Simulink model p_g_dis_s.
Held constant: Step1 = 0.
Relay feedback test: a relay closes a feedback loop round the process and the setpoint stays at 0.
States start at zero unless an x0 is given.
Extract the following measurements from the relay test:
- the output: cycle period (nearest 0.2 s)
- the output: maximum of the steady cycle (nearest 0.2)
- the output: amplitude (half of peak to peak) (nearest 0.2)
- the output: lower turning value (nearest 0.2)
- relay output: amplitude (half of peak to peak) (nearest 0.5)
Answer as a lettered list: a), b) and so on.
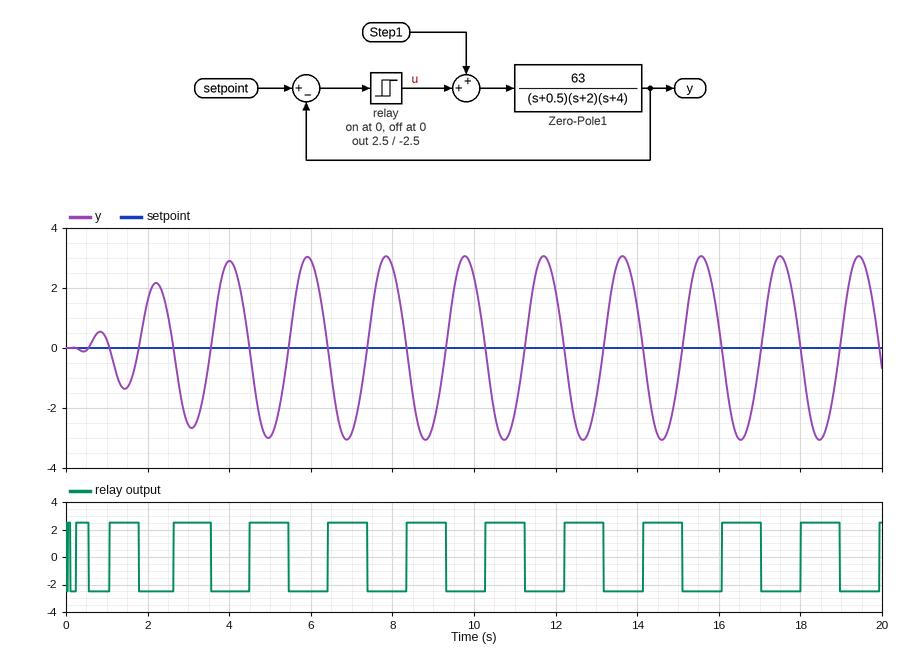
a) 2.0 s
b) 3.0
c) 3.0
d) -3.0
e) 2.5
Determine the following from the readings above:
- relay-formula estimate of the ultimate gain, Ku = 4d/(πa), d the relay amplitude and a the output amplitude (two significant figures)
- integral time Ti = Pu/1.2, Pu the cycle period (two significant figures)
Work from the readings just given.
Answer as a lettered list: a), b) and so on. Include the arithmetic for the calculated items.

a) 4 × 2.5 / (π × 3) = 1.1
b) 2 / 1.2 = 1.7 s
